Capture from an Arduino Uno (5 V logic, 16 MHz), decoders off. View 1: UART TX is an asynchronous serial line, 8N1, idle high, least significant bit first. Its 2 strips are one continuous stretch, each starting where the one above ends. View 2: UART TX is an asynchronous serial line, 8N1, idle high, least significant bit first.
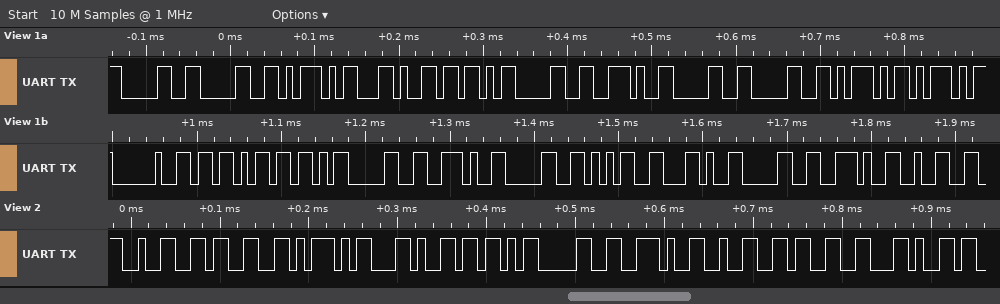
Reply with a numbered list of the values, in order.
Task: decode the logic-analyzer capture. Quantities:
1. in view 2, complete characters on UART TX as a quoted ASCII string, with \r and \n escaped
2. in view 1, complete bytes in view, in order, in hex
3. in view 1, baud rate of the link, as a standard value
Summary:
1. "23],[0.23,"
2. 0x30 0x30 0x5D 0x2C 0x5B 0x30 0x2E 0x30 0x30 0x5D 0x5D 0x20 0x5B 0x5B 0x30 0x2E 0x30 0x35 0x2C 0x30 0x2E 0x32
3. 115200 baud
